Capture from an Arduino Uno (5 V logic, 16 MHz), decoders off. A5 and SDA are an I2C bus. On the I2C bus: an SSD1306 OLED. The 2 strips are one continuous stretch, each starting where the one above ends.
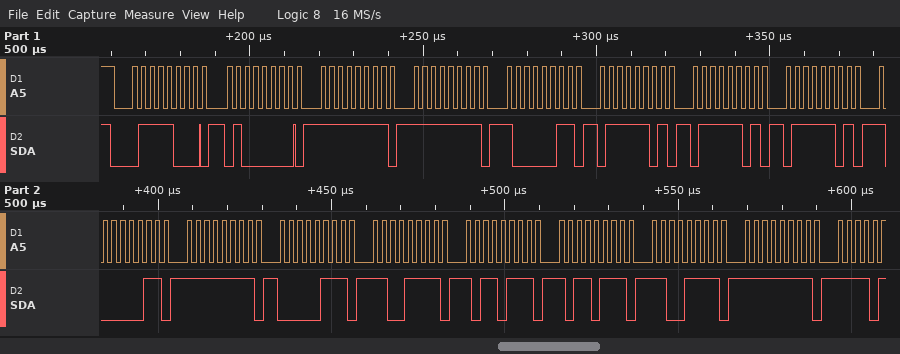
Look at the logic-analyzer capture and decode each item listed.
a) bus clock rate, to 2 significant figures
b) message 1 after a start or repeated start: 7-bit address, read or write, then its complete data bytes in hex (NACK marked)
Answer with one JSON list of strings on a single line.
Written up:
["400 kHz", "0x3C write: 40 FF FF 83 7D 7D 7D 83 FF 07 CF B7 B7 CF FF"]
